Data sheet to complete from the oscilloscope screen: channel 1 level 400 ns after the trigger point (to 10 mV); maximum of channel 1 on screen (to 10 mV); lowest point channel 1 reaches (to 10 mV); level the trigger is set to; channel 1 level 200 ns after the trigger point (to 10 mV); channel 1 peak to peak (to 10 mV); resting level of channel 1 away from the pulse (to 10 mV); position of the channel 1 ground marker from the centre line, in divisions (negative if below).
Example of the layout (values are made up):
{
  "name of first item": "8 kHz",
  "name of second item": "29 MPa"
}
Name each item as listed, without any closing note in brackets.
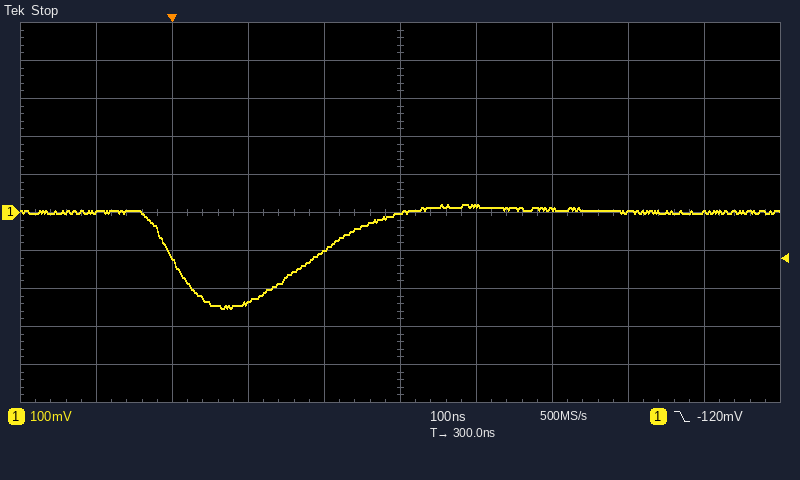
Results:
{
  "channel 1 level 400 ns after the trigger point": "20 mV",
  "maximum of channel 1 on screen": "20 mV",
  "lowest point channel 1 reaches": "-250 mV",
  "level the trigger is set to": "-120 mV",
  "channel 1 level 200 ns after the trigger point": "-100 mV",
  "channel 1 peak to peak": "270 mV",
  "resting level of channel 1 away from the pulse": "0 mV",
  "position of the channel 1 ground marker from the centre line, in divisions": "0.0 div"
}
